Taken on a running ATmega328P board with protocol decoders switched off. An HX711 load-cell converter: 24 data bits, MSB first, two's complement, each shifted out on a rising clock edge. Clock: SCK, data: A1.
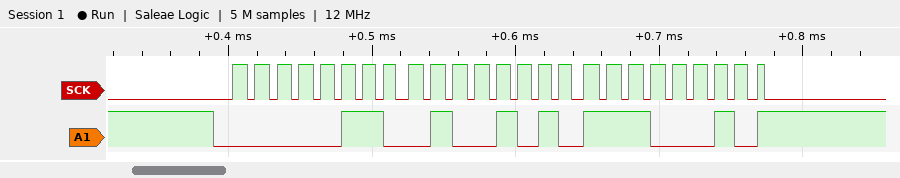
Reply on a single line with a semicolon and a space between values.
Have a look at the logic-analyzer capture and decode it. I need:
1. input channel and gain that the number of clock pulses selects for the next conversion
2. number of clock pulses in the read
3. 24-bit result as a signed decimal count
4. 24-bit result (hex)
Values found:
channel A, gain 128; 25; 412386; 0x064AE2
